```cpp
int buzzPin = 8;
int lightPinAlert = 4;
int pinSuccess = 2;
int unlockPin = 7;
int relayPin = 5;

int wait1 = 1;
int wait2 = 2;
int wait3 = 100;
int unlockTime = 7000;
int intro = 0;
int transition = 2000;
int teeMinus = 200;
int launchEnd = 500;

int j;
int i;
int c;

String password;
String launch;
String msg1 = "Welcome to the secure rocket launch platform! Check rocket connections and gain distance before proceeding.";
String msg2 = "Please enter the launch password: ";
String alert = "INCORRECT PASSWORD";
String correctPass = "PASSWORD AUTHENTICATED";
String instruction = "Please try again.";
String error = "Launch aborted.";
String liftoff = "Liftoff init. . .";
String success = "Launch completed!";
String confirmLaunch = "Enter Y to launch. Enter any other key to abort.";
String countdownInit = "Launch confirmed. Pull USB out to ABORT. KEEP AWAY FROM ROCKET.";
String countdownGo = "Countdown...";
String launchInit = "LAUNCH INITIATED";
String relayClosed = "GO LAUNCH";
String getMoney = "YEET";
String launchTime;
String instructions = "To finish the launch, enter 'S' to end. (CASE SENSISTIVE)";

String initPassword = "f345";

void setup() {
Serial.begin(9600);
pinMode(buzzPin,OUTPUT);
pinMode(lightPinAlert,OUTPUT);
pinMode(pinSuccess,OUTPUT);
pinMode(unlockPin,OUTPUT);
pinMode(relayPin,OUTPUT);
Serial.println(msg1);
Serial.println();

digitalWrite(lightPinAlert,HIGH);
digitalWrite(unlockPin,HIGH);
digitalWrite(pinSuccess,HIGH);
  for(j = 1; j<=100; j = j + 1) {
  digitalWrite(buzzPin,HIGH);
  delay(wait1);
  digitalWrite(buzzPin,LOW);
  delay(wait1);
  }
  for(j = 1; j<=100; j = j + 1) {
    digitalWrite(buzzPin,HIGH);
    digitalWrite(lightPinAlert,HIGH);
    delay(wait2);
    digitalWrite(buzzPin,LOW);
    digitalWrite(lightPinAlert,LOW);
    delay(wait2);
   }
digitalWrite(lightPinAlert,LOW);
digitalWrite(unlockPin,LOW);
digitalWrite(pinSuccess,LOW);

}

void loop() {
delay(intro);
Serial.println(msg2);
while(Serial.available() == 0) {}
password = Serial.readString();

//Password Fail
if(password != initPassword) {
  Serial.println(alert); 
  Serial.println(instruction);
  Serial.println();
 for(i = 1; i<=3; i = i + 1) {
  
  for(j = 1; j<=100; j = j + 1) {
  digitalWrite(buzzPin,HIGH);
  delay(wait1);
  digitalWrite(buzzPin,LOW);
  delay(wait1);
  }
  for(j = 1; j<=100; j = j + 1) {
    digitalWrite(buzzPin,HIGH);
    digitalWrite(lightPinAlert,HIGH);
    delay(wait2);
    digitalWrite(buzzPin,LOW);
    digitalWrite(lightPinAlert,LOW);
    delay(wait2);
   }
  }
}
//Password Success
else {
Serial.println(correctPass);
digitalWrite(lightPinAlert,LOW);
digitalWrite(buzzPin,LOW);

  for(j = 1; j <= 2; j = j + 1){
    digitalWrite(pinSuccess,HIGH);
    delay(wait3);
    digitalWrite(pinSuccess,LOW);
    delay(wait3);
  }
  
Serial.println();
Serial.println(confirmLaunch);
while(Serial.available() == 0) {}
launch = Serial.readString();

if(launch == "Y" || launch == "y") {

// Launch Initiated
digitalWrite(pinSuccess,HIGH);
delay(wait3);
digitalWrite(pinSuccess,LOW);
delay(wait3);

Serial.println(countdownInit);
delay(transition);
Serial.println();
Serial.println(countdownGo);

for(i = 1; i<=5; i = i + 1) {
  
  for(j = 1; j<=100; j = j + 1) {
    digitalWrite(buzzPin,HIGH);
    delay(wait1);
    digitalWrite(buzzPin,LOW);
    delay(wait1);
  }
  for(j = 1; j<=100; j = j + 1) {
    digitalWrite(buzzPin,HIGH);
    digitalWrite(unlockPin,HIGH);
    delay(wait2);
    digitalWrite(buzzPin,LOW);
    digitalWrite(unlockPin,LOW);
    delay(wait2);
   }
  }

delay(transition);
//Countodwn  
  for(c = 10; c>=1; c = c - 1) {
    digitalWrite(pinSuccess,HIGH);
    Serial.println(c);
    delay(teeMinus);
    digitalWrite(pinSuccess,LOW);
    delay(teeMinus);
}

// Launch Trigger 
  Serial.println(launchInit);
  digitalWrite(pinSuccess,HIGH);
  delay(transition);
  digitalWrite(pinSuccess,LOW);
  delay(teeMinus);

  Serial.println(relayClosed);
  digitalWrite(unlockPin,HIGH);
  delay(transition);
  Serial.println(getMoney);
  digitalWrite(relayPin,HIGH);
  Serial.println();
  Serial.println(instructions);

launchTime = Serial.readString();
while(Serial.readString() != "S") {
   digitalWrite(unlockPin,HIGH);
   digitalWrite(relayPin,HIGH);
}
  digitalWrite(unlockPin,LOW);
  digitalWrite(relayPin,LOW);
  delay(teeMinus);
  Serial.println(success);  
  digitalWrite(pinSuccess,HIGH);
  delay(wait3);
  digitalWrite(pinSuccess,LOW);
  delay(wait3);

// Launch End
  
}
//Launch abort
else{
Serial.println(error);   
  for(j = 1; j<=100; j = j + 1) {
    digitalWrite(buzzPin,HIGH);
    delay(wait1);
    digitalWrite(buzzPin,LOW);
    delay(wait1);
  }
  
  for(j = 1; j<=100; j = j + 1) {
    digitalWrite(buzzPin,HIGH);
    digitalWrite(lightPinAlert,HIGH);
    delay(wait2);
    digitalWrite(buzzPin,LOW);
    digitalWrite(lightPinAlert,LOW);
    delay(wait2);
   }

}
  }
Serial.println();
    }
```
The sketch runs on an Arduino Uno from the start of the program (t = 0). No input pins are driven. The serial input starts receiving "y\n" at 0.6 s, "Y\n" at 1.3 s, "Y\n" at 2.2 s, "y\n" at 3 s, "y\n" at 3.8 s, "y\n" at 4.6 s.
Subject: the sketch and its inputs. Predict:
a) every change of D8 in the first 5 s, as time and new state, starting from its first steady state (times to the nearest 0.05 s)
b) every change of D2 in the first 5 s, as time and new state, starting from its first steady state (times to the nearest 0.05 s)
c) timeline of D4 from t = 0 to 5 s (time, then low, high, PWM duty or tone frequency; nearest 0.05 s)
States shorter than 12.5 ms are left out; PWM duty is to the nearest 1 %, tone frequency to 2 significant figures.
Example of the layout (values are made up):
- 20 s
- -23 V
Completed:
- 0 s low; 0.05 s tone 330 Hz; 0.65 s low
- 0 s low; 0.05 s high; 0.65 s low
- 0 s low; 0.05 s high; 0.25 s tone 250 Hz; 0.65 s low
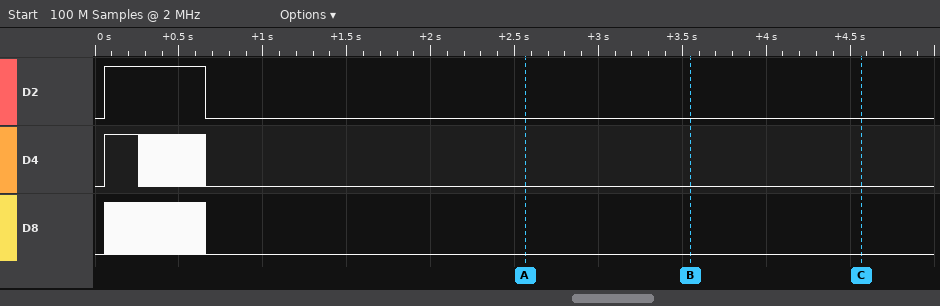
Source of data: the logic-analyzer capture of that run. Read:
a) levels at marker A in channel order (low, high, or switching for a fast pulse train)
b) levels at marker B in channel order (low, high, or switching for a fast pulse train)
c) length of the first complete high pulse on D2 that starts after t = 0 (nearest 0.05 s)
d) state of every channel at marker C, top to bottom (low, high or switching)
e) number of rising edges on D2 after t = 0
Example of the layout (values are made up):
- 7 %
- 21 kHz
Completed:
- D2 low, D4 low, D8 low
- D2 low, D4 low, D8 low
- 0.60 s
- D2 low, D4 low, D8 low
- 1
